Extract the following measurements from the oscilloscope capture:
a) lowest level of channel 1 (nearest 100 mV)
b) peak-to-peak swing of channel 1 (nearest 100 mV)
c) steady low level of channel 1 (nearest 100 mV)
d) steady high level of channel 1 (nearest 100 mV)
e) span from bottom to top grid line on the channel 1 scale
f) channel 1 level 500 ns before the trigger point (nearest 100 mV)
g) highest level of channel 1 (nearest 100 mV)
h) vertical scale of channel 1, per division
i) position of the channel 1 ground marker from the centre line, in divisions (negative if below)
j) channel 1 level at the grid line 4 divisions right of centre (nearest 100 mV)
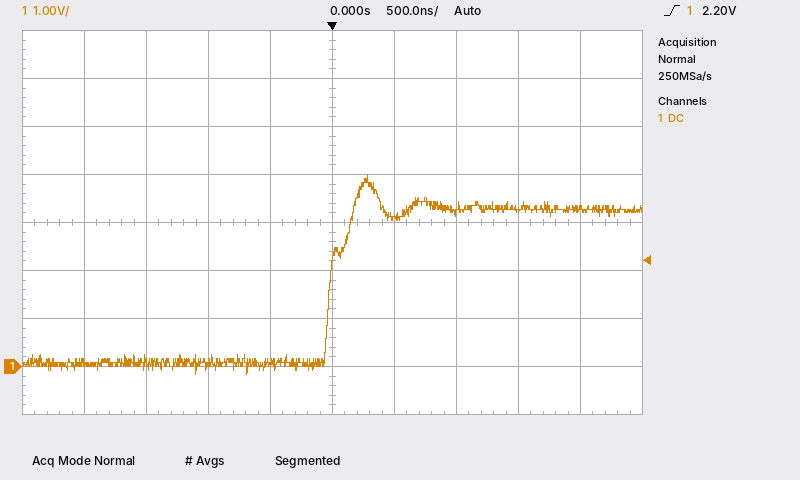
-200 mV
4.2 V
100 mV
3.3 V
8 V
100 mV
4.0 V
1 V
-3.0 div
3.3 V
